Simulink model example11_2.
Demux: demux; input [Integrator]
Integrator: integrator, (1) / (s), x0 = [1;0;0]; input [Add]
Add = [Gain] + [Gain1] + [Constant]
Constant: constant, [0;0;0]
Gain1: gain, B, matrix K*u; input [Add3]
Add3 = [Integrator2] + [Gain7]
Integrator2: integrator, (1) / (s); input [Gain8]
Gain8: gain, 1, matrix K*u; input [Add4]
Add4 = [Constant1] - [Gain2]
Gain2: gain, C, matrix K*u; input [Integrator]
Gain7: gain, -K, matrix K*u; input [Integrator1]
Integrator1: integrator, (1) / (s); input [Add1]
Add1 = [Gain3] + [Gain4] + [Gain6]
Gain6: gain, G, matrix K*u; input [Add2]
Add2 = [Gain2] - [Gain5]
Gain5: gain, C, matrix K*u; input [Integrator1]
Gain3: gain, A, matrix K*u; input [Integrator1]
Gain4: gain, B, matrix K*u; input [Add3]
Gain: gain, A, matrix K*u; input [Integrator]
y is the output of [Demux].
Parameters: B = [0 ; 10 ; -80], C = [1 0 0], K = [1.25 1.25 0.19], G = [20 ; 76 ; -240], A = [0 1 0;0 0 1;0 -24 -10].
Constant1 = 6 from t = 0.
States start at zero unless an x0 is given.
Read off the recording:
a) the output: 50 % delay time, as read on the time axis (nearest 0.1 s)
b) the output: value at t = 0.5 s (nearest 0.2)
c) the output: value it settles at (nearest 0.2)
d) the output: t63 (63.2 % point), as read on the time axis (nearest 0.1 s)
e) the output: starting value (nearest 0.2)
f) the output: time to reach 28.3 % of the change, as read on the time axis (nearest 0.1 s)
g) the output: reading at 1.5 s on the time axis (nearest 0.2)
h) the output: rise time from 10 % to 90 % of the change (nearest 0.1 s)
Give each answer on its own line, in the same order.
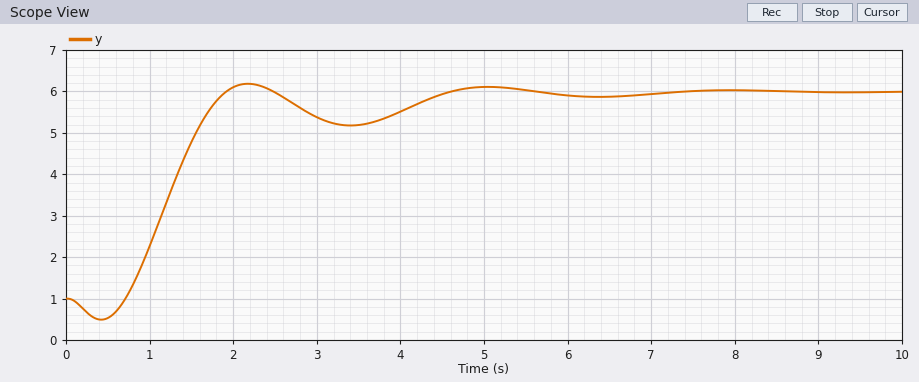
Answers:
1.2 s
0.6
6.0
1.4 s
1.0
1.0 s
4.8
0.9 s
